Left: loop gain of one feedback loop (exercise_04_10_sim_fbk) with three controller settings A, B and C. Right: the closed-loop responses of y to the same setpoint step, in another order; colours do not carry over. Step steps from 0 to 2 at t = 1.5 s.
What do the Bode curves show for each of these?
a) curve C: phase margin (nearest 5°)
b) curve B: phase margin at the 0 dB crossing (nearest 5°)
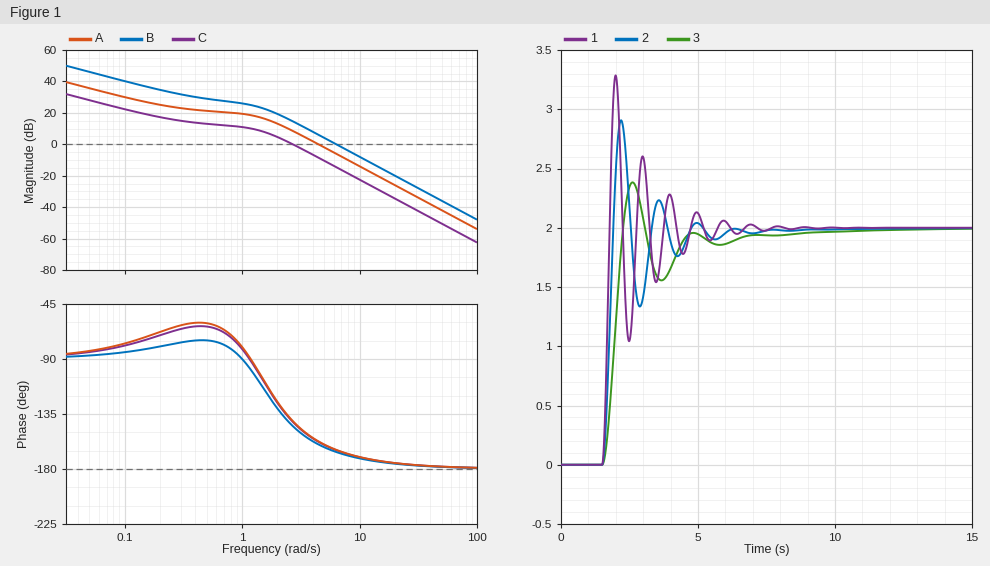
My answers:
40°
15°
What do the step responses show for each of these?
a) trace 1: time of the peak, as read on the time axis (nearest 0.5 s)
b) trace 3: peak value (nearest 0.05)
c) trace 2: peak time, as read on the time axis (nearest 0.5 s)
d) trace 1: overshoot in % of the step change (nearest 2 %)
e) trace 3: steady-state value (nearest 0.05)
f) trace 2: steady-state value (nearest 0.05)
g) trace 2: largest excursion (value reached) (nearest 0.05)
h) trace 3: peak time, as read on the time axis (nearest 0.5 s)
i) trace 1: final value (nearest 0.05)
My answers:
2.0 s
2.40
2.0 s
64 %
2.00
2.00
2.90
2.5 s
2.00
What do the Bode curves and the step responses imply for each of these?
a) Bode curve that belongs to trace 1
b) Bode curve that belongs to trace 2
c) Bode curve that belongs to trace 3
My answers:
B
A
C
